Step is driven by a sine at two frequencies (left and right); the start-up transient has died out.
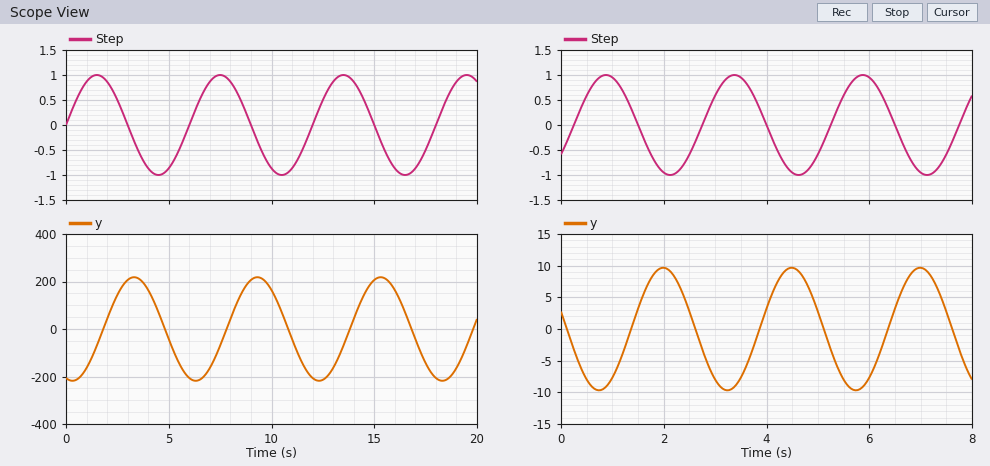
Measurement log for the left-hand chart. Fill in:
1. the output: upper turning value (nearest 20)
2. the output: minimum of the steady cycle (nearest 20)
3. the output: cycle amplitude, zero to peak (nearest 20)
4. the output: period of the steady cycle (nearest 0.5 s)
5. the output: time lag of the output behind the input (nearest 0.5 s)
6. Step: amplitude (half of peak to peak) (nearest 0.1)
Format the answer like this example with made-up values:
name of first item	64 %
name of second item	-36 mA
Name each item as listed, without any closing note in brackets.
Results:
the output: upper turning value	220
the output: minimum of the steady cycle	-220
the output: cycle amplitude, zero to peak	220
the output: period of the steady cycle	6.0 s
the output: time lag of the output behind the input	2.0 s
Step: amplitude (half of peak to peak)	1.0
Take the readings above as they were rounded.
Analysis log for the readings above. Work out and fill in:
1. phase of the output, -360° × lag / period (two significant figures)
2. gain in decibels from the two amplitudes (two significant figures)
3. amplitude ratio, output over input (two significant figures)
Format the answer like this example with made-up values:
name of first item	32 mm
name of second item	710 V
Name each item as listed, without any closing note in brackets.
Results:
phase of the output, -360° × lag / period	-120°
gain in decibels from the two amplitudes	47 dB
amplitude ratio, output over input	220
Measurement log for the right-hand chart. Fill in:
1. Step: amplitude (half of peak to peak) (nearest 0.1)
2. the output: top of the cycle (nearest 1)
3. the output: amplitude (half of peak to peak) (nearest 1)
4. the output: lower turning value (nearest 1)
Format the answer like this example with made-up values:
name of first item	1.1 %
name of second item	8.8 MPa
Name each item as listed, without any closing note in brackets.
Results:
Step: amplitude (half of peak to peak)	1.0
the output: top of the cycle	10
the output: amplitude (half of peak to peak)	10
the output: lower turning value	-10
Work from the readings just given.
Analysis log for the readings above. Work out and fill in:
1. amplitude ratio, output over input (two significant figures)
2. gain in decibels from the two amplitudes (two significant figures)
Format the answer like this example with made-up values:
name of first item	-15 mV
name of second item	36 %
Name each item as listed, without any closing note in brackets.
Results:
amplitude ratio, output over input	10
gain in decibels from the two amplitudes	20 dB
